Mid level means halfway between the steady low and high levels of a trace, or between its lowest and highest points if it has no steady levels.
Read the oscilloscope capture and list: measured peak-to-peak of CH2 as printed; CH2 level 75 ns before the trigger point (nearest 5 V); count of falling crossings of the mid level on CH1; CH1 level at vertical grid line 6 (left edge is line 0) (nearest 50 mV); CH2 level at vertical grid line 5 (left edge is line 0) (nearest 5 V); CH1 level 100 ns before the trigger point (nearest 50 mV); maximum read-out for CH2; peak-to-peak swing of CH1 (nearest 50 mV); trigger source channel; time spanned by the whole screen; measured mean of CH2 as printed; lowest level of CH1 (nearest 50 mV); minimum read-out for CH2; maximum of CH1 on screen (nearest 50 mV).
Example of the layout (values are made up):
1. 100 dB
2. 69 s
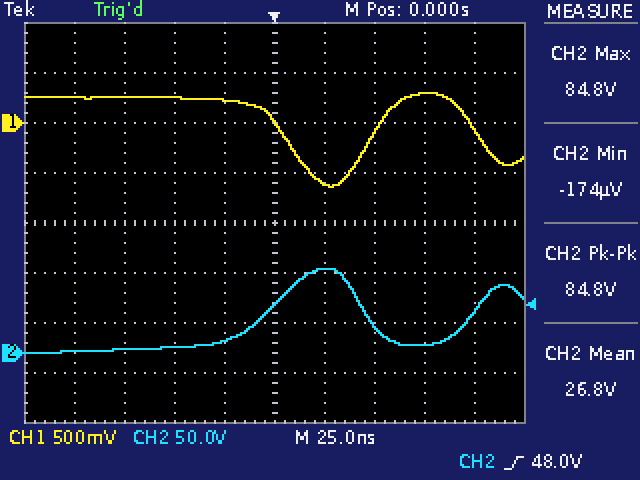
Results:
1. 84.8 V
2. 5 V
3. 2
4. -600 mV
5. 50 V
6. 250 mV
7. 84.8 V
8. 950 mV
9. CH2
10. 250 ns
11. 26.8 V
12. -650 mV
13. -174 µV
14. 300 mV
